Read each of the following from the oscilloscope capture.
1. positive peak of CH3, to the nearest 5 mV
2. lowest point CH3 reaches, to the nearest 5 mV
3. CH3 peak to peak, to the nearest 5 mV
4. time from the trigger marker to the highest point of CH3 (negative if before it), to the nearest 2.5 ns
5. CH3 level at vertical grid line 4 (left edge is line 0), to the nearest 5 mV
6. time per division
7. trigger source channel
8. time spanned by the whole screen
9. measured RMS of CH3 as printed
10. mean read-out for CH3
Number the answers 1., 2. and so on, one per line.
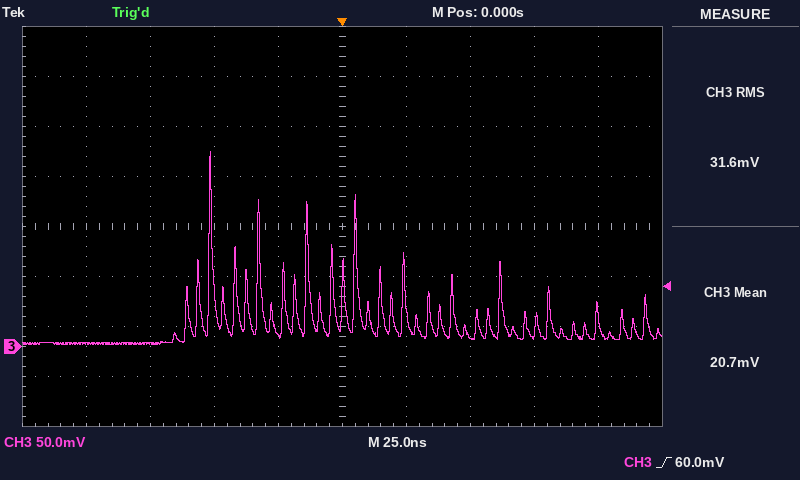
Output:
1. 195 mV
2. 0 mV
3. 195 mV
4. -52.5 ns
5. 15 mV
6. 25 ns
7. CH3
8. 250 ns
9. 31.6 mV
10. 20.7 mV
